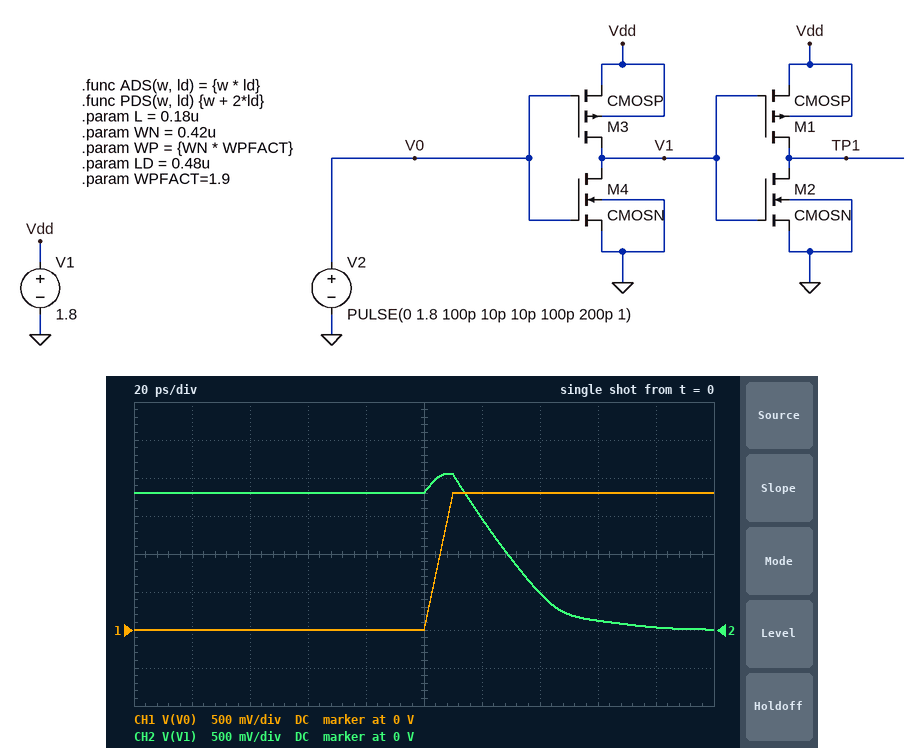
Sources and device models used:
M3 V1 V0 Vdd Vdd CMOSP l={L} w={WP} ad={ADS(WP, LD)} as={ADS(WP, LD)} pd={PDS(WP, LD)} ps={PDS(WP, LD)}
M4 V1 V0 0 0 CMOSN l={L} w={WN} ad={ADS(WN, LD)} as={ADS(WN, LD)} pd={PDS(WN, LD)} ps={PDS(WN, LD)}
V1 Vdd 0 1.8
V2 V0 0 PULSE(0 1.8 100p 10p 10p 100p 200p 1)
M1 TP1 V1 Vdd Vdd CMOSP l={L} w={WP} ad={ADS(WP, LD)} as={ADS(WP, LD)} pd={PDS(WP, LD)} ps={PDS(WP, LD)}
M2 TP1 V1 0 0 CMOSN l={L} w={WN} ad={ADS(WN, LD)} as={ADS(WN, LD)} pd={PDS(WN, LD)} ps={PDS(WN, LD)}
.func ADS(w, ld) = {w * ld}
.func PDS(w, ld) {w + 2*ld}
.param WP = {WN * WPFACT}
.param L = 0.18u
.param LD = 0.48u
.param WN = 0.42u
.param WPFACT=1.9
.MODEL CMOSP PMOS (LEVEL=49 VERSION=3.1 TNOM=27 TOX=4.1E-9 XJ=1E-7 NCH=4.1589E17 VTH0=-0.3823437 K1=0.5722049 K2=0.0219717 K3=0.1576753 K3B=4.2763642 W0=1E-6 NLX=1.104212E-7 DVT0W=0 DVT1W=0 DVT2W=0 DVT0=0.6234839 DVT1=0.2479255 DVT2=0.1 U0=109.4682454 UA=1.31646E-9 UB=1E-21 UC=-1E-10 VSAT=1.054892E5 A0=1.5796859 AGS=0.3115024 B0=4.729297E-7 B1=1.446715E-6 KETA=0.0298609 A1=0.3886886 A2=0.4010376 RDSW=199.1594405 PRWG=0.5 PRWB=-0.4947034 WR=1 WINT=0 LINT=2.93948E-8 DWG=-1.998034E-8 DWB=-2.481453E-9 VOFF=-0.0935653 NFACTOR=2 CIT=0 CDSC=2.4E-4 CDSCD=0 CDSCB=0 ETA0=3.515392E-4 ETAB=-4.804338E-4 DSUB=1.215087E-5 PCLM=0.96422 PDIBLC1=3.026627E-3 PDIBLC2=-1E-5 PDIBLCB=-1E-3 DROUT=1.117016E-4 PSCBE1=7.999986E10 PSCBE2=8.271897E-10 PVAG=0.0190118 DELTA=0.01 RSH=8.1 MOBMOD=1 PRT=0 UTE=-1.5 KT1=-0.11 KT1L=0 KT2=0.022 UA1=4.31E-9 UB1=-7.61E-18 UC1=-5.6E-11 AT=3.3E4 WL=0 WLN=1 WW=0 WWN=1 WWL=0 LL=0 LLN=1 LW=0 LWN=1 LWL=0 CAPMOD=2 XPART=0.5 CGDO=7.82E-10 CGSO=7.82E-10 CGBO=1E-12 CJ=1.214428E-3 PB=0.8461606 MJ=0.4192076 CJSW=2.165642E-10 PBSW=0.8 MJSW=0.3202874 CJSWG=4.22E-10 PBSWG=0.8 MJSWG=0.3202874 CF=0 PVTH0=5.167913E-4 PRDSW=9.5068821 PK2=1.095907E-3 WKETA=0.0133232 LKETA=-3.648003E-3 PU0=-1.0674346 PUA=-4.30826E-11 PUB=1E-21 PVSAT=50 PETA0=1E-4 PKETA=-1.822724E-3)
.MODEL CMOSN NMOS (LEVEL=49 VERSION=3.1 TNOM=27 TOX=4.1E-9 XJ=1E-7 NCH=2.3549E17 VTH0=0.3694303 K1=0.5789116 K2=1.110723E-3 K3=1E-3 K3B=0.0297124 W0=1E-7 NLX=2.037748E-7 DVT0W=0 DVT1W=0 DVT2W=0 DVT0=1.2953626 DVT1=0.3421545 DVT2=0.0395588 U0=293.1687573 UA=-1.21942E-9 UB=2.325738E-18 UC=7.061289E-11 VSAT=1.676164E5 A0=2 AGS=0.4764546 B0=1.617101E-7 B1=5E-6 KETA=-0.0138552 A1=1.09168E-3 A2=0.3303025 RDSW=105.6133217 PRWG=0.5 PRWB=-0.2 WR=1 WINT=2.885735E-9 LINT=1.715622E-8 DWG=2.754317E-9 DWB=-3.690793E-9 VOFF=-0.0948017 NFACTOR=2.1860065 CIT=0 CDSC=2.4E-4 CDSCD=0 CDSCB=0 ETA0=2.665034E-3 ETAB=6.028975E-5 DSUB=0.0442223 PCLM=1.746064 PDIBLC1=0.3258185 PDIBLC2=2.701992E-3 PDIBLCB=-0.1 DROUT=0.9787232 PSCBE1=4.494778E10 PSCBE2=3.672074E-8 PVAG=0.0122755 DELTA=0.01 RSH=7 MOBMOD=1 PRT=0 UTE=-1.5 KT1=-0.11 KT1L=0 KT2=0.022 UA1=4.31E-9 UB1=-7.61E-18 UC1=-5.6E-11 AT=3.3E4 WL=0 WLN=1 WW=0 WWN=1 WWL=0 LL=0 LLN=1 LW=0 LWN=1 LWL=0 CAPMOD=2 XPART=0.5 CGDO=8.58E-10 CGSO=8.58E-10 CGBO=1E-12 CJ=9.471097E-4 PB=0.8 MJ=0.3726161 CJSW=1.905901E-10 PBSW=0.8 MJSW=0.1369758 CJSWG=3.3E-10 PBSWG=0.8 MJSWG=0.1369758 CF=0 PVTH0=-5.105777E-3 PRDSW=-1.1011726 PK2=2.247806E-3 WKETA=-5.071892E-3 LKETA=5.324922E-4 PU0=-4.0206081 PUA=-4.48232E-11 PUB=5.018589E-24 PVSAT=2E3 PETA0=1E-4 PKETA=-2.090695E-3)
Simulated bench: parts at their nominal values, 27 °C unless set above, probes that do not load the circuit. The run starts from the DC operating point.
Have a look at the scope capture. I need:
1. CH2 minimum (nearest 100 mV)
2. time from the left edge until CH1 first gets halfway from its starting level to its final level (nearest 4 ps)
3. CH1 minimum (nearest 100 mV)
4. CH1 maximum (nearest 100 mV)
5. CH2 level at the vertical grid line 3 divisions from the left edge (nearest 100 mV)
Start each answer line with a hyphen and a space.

- 0 V
- 104 ps
- 0 V
- 1.8 V
- 1.8 V
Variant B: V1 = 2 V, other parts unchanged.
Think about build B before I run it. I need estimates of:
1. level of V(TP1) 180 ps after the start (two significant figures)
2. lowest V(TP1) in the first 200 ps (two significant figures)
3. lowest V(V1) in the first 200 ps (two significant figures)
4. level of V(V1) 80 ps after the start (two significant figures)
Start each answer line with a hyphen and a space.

- 1.9 V
- -110 mV
- 4.9 mV
- 2.0 V
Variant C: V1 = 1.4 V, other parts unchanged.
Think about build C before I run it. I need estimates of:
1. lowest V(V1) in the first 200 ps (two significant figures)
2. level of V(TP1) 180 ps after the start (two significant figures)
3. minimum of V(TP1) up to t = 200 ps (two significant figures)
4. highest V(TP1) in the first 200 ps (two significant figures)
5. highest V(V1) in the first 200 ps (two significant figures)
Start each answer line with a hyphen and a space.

- 7.3 mV
- 1.3 V
- -190 mV
- 1.4 V
- 1.7 V
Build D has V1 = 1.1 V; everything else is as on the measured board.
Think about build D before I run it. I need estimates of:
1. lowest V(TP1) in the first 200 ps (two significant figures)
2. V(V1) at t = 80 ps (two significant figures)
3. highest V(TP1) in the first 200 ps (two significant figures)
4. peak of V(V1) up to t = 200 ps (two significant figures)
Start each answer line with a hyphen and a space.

- -260 mV
- 1.1 V
- 1.0 V
- 1.4 V
